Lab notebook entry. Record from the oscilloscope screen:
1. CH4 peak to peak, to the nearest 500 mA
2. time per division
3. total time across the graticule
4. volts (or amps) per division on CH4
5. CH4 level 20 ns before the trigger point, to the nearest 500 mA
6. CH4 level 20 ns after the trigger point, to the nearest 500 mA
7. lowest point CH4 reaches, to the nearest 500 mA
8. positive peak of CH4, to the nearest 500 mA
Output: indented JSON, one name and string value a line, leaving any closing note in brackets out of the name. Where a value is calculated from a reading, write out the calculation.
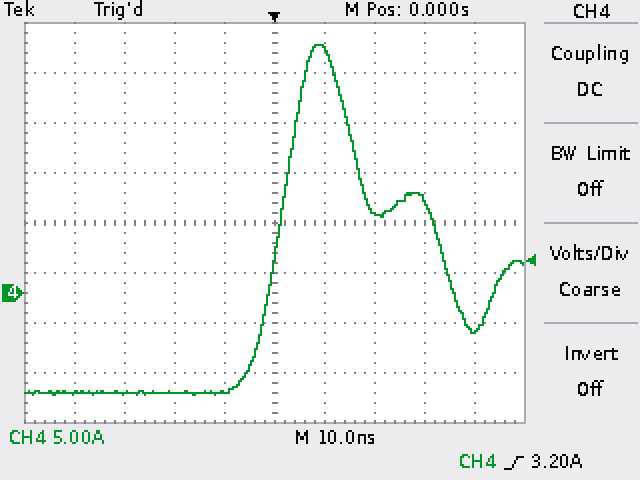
{
  "CH4 peak to peak, to the nearest 500 mA": "25.0 A − (-10.0 A) = 35.0 A",
  "time per division": "10 ns",
  "total time across the graticule": "100 ns",
  "volts (or amps) per division on CH4": "5 A",
  "CH4 level 20 ns before the trigger point, to the nearest 500 mA": "-10.0 A",
  "CH4 level 20 ns after the trigger point, to the nearest 500 mA": "8.0 A",
  "lowest point CH4 reaches, to the nearest 500 mA": "-10.0 A",
  "positive peak of CH4, to the nearest 500 mA": "25.0 A"
}
